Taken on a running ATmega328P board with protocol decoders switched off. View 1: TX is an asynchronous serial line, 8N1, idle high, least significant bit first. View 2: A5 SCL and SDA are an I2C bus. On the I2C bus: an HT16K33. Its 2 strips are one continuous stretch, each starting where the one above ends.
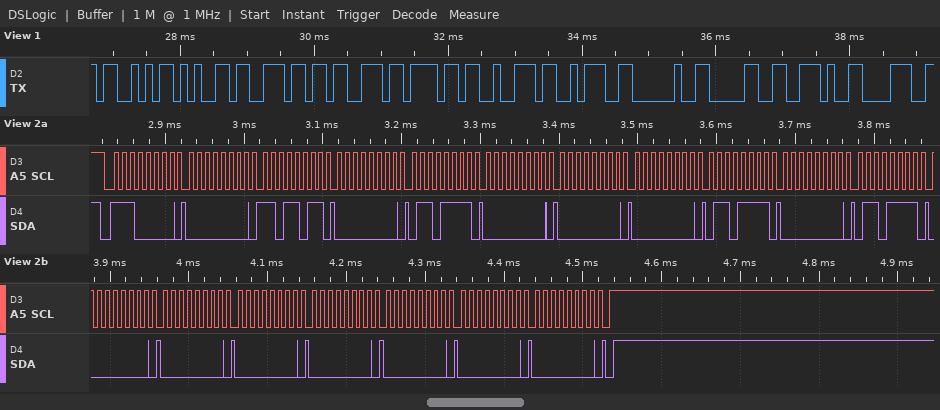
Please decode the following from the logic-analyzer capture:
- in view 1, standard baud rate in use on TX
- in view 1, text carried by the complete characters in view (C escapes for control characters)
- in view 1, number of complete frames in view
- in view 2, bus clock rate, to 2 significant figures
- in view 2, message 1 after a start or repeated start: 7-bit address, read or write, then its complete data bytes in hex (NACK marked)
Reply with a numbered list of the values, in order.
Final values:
1. 9600 baud
2. "Sensor: 0.8"
3. 11
4. 100 kHz
5. 0x70 write: 00 DB 00 6F 00 00 00 6F 00 6F 00 00 00 00 00 00 00
